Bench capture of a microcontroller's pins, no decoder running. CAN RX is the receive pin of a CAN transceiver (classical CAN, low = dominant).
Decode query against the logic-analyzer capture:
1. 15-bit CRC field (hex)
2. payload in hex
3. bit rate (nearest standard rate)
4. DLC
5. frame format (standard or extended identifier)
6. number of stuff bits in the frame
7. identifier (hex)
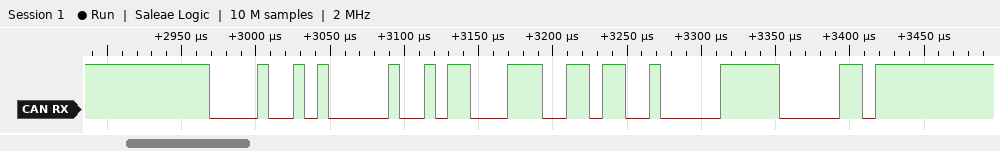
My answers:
0x20F0
C7 36
125 kbit/s
2
standard
4
0x094
